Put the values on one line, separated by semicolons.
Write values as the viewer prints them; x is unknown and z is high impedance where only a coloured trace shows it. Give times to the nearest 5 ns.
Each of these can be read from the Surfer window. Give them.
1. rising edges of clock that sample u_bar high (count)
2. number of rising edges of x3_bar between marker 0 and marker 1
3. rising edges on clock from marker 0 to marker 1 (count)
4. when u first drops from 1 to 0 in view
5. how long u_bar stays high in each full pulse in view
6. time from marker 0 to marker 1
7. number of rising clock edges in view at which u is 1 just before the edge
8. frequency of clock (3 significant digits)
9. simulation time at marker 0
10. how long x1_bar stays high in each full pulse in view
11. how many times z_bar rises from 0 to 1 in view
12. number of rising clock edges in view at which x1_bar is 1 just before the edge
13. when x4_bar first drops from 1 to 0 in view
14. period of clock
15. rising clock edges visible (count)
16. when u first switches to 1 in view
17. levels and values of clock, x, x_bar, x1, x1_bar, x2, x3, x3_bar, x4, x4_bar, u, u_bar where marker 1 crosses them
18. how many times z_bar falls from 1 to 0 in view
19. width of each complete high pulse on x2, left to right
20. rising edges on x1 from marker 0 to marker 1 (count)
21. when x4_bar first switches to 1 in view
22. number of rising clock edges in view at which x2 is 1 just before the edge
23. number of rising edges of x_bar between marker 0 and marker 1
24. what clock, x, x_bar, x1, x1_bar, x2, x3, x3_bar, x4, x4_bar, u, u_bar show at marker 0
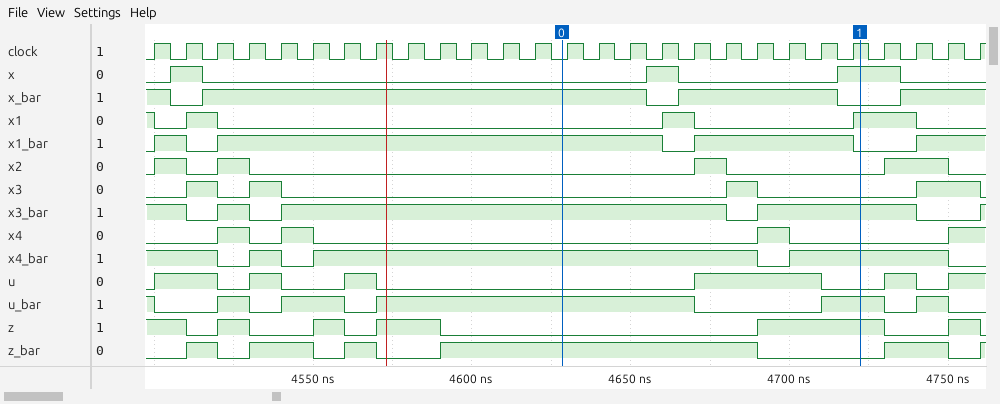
17; 1; 10; 4520 ns; 10 ns, 20 ns, 100 ns, 20 ns, 10 ns; 95 ns; 10; 100 MHz; 4630 ns; 10 ns, 140 ns, 50 ns; 6; 22; 4520 ns; 10 ns; 27; 4500 ns; clock=1, x=1, x_bar=0, x1=1, x1_bar=0, x2=0, x3=0, x3_bar=1, x4=0, x4_bar=1, u=0, u_bar=1; 5; 10 ns, 10 ns, 10 ns, 20 ns; 2; 4530 ns; 5; 1; clock=0, x=0, x_bar=1, x1=0, x1_bar=1, x2=0, x3=0, x3_bar=1, x4=0, x4_bar=1, u=0, u_bar=1
